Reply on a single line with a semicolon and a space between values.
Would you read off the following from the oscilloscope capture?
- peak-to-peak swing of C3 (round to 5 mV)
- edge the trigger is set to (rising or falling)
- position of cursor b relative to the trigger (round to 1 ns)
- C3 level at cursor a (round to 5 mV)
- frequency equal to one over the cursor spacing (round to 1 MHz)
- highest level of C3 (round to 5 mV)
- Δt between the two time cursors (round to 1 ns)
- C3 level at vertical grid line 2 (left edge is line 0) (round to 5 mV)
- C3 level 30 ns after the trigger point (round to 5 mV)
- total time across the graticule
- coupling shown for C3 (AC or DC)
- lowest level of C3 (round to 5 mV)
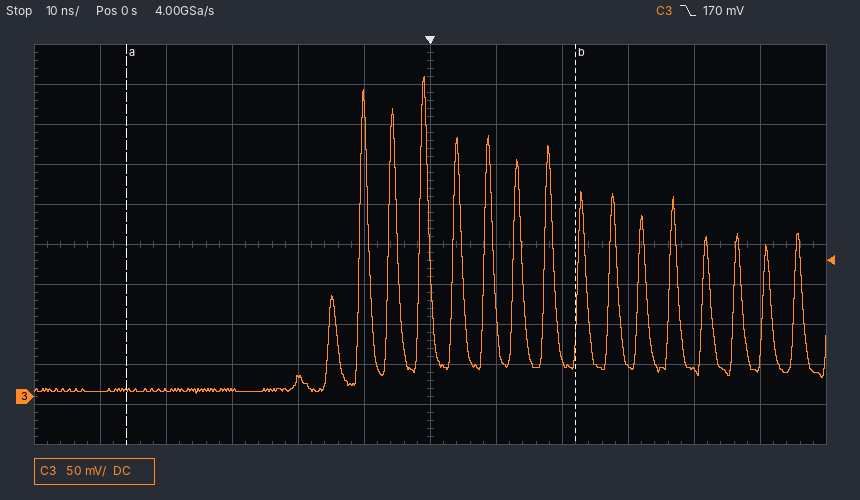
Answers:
395 mV; falling; +22 ns; 10 mV; 15 MHz; 400 mV; 68 ns; 10 mV; 40 mV; 120 ns; DC; 5 mV
